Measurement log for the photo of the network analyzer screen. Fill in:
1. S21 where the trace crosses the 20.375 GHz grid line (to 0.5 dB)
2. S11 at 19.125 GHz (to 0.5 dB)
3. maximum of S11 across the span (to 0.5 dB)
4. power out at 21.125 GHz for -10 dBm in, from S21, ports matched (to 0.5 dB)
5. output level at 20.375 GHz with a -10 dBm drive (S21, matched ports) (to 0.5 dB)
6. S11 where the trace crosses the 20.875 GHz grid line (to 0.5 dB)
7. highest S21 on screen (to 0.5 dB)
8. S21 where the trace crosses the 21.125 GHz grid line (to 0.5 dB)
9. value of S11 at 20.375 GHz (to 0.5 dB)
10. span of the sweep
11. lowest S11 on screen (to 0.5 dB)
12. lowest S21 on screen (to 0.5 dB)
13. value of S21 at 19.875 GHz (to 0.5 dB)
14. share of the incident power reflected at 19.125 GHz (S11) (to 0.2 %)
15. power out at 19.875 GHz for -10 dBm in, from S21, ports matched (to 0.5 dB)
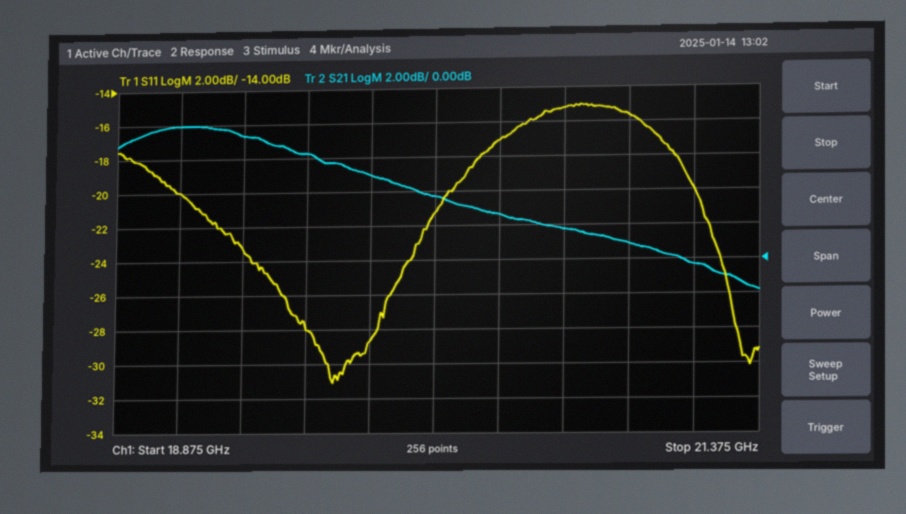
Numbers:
2.5 dB
-20.0 dB
-15.0 dB
-10.5 dBm
-7.5 dBm
-15.5 dB
8.0 dB
-0.5 dB
-17.0 dB
2.5 GHz
-31.0 dB
-2.0 dB
5.0 dB
1.0 %
-5.0 dBm
